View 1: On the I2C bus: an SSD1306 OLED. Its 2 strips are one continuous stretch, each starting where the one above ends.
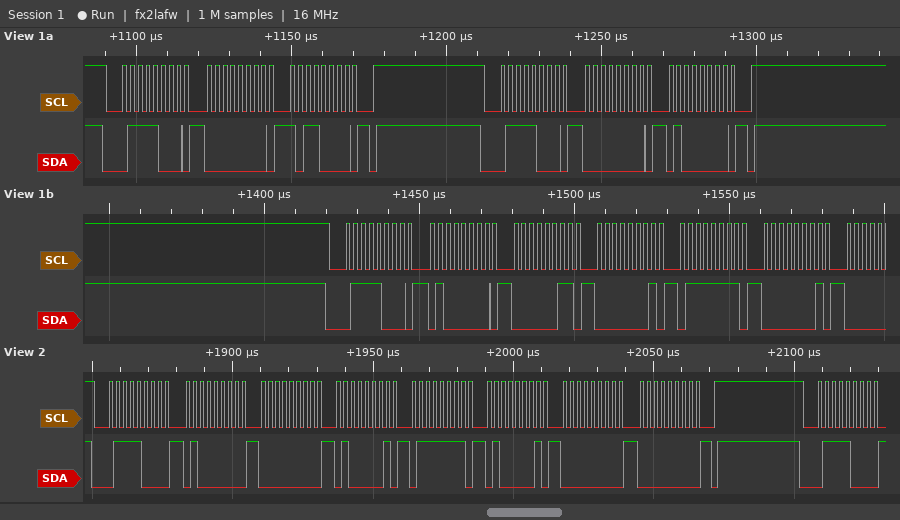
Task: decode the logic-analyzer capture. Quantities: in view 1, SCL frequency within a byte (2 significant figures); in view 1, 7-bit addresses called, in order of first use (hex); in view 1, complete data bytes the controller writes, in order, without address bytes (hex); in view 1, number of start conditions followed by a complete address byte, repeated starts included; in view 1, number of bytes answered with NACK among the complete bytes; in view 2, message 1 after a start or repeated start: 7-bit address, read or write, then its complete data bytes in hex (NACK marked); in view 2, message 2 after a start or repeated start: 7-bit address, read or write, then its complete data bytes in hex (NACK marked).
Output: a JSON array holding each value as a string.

["400 kHz", "0x3C", "00 B0 00 40 40 03 01 7F 01", "3", "0", "0x3C write: 40 00 41 7F 41 00 00", "0x3C write"]
